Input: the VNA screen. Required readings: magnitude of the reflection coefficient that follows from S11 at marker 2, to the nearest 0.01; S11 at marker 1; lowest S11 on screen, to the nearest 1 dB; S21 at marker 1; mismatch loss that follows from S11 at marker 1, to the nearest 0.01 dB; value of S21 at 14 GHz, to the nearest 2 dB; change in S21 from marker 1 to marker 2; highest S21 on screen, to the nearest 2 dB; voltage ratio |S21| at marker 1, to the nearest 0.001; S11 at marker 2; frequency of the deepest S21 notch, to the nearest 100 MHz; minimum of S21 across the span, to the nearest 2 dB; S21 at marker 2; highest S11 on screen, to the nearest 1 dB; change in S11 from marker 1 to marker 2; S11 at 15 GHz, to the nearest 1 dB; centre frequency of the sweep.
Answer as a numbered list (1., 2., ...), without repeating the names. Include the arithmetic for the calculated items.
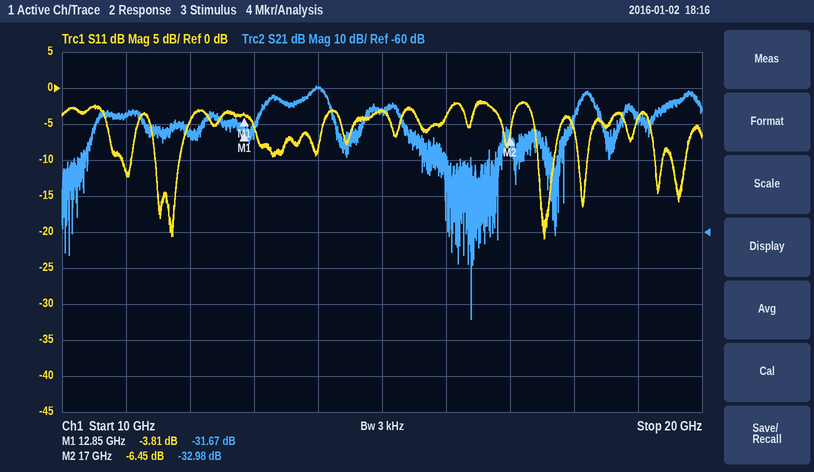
1. 10^(-6.45/20) ≈ 0.48
2. -3.81 dB
3. -21 dB
4. -31.67 dB
5. −10 log10(1 − 10^(-3.81/10)) ≈ 2.34 dB
6. -20 dB
7. -32.98 − (-31.67) = -1.31 dB
8. -20 dB
9. 10^(-31.67/20) ≈ 0.026
10. -6.45 dB
11. 16.4 GHz
12. -84 dB
13. -32.98 dB
14. -2 dB
15. -6.45 − (-3.81) = -2.64 dB
16. -3 dB
17. 15 GHz
